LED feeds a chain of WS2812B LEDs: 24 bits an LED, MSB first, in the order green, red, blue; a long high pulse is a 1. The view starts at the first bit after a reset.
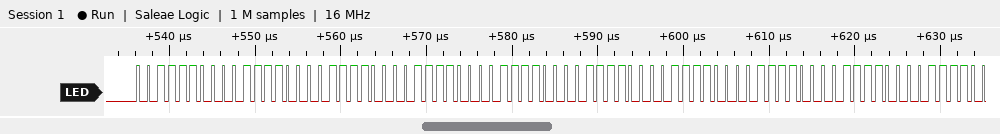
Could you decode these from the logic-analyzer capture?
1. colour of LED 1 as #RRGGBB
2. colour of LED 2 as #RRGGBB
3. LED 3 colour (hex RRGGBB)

#3C3C3C
#3C3C3C
#3C3C3C
